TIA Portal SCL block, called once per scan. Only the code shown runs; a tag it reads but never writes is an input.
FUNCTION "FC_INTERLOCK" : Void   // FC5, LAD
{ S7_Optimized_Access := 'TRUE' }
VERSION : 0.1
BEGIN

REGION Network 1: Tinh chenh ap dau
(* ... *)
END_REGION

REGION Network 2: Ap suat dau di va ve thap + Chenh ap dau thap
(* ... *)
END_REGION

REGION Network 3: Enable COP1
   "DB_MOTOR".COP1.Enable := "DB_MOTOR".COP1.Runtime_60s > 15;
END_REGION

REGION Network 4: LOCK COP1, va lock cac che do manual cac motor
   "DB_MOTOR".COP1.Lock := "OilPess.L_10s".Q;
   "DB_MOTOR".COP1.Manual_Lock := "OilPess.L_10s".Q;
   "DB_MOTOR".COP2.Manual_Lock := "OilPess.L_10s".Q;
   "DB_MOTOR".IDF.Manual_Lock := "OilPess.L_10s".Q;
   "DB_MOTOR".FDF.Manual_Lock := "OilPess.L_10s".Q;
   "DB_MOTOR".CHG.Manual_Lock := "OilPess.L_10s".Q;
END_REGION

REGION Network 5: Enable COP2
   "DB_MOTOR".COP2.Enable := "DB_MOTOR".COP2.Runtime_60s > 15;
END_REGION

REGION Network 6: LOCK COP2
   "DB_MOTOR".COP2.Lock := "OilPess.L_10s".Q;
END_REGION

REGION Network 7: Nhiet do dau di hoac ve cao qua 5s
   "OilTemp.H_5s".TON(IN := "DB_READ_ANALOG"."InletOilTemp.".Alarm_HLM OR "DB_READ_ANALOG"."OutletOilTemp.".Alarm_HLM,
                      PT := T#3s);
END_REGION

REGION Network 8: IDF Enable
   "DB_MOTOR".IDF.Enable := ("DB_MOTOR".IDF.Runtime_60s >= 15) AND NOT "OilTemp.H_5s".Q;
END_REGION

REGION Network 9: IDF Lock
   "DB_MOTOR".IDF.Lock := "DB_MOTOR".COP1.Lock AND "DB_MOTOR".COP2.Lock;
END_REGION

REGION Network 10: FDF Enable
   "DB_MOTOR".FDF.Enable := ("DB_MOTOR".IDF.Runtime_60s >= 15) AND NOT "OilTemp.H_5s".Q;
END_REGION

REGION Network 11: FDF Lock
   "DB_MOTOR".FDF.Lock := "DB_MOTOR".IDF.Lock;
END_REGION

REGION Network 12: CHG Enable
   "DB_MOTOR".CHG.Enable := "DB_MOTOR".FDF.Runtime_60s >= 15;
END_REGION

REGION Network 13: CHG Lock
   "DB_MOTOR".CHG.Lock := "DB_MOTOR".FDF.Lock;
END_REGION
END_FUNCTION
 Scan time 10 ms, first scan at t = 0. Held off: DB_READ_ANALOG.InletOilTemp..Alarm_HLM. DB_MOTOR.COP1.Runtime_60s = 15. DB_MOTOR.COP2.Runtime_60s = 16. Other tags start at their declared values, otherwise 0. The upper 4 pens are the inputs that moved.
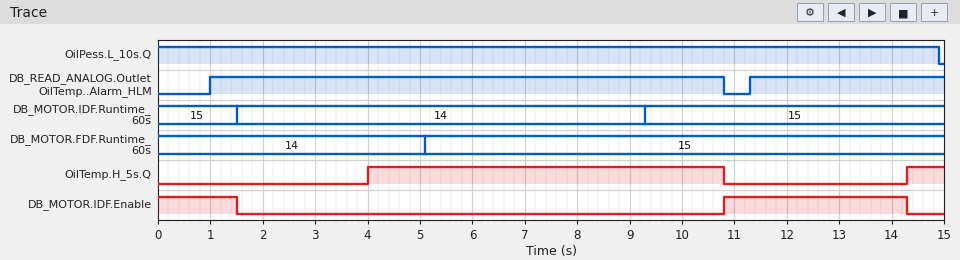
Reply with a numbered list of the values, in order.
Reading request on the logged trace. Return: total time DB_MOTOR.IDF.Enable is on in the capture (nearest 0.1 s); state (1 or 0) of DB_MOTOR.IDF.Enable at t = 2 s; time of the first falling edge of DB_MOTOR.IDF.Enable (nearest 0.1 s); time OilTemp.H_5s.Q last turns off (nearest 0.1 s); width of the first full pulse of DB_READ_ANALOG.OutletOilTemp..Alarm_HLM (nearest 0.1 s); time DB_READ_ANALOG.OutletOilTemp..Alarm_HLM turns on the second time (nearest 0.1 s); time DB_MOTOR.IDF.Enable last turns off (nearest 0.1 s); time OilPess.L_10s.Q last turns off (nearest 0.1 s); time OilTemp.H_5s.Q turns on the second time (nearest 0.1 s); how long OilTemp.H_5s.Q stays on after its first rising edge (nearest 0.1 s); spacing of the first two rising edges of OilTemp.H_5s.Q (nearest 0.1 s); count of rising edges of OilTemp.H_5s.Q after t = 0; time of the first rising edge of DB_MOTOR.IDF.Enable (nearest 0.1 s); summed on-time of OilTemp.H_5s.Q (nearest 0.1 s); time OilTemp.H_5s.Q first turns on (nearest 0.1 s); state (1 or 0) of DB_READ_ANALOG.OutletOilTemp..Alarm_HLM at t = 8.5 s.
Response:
1. 5.0 s
2. 0
3. 1.5 s
4. 10.8 s
5. 9.8 s
6. 11.3 s
7. 14.3 s
8. 14.9 s
9. 14.3 s
10. 6.8 s
11. 10.3 s
12. 2
13. 10.8 s
14. 7.5 s
15. 4.0 s
16. 1
